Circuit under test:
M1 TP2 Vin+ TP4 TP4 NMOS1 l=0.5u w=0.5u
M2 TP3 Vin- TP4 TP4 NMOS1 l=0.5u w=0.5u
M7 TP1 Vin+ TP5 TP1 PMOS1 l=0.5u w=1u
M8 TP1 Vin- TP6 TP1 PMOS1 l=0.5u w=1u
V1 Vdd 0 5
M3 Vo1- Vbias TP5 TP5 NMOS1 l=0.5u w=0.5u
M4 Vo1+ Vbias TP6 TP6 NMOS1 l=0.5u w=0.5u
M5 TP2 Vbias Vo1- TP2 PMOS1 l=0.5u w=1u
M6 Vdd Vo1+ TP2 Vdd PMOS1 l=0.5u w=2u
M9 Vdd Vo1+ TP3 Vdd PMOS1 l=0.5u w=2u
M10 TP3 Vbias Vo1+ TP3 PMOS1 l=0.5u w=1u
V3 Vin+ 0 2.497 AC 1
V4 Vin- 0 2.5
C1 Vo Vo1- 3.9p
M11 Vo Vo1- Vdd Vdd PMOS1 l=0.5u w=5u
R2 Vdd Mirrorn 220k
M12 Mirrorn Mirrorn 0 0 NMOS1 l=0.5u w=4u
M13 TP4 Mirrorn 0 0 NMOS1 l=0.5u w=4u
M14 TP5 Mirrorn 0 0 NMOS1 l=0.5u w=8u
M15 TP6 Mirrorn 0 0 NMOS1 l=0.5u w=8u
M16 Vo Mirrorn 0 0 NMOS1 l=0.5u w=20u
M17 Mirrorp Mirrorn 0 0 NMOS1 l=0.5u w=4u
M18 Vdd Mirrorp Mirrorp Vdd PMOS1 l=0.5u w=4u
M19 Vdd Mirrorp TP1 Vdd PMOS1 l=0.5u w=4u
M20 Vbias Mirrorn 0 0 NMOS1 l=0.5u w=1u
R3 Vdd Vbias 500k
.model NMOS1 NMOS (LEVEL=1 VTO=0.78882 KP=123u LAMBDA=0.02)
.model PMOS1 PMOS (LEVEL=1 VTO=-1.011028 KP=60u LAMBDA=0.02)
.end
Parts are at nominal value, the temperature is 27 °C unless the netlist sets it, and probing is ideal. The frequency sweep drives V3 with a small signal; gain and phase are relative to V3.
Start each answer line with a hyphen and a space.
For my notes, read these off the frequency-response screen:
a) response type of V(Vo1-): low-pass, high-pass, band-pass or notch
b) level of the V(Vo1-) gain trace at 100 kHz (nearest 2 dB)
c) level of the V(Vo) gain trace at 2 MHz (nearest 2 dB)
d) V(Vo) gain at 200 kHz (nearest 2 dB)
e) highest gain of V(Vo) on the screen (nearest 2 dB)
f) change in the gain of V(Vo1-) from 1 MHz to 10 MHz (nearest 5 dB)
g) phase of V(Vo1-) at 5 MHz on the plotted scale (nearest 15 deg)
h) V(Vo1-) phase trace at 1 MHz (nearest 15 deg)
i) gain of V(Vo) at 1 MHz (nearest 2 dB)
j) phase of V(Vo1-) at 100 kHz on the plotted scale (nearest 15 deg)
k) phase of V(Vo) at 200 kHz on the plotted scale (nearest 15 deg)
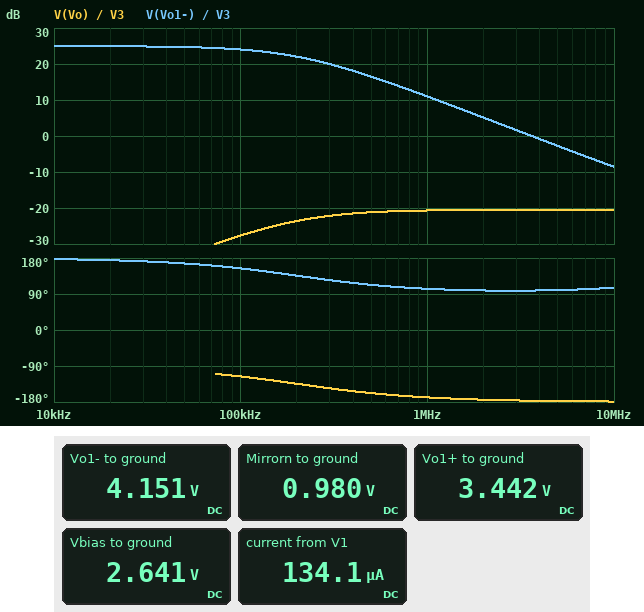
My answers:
- low-pass
- 24 dB
- -20 dB
- -24 dB
- -20 dB
- -20 dB
- 105 deg
- 105 deg
- -20 dB
- 150 deg
- -135 deg
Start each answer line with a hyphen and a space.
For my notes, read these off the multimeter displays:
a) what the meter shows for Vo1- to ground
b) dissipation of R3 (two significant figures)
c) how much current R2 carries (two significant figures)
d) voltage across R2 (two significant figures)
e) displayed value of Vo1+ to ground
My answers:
- 4.151 V
- 11 µW
- 18 µA
- 4.0 V
- 3.442 V
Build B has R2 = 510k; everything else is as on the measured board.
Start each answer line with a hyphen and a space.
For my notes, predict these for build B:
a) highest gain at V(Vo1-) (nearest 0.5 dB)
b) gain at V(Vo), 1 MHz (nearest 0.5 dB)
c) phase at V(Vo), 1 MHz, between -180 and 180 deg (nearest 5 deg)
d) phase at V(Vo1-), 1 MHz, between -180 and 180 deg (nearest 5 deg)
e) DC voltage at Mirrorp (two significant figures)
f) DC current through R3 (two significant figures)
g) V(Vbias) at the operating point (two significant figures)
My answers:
- -22.0 dB
- -61.0 dB
- -75 deg
- 170 deg
- 3.8 V
- 2.1 µA
- 3.9 V
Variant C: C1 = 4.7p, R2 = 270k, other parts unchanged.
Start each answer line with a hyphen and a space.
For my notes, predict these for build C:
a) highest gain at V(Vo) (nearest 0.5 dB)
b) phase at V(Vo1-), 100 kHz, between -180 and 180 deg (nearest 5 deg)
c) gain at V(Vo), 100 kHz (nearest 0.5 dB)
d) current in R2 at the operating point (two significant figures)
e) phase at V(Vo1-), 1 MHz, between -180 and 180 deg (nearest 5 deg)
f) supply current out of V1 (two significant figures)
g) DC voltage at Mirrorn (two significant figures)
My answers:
- -22.0 dB
- 135 deg
- -25.0 dB
- 15 µA
- 100 deg
- 110 µA
- 960 mV
